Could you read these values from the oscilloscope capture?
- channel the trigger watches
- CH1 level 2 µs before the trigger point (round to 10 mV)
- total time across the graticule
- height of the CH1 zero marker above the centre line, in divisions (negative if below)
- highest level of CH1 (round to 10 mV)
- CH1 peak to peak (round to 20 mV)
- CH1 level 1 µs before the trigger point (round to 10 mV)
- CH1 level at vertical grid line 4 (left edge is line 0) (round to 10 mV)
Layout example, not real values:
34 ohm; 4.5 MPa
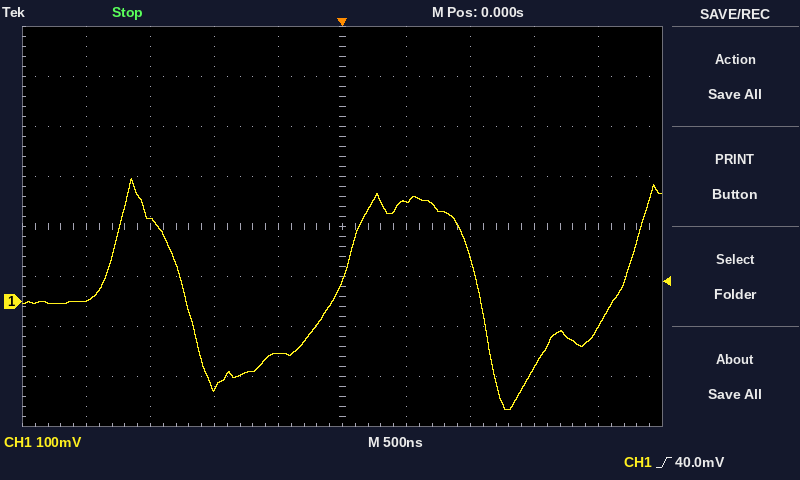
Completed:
CH1; 0 mV; 5 µs; -1.5 div; 250 mV; 460 mV; -170 mV; -100 mV
